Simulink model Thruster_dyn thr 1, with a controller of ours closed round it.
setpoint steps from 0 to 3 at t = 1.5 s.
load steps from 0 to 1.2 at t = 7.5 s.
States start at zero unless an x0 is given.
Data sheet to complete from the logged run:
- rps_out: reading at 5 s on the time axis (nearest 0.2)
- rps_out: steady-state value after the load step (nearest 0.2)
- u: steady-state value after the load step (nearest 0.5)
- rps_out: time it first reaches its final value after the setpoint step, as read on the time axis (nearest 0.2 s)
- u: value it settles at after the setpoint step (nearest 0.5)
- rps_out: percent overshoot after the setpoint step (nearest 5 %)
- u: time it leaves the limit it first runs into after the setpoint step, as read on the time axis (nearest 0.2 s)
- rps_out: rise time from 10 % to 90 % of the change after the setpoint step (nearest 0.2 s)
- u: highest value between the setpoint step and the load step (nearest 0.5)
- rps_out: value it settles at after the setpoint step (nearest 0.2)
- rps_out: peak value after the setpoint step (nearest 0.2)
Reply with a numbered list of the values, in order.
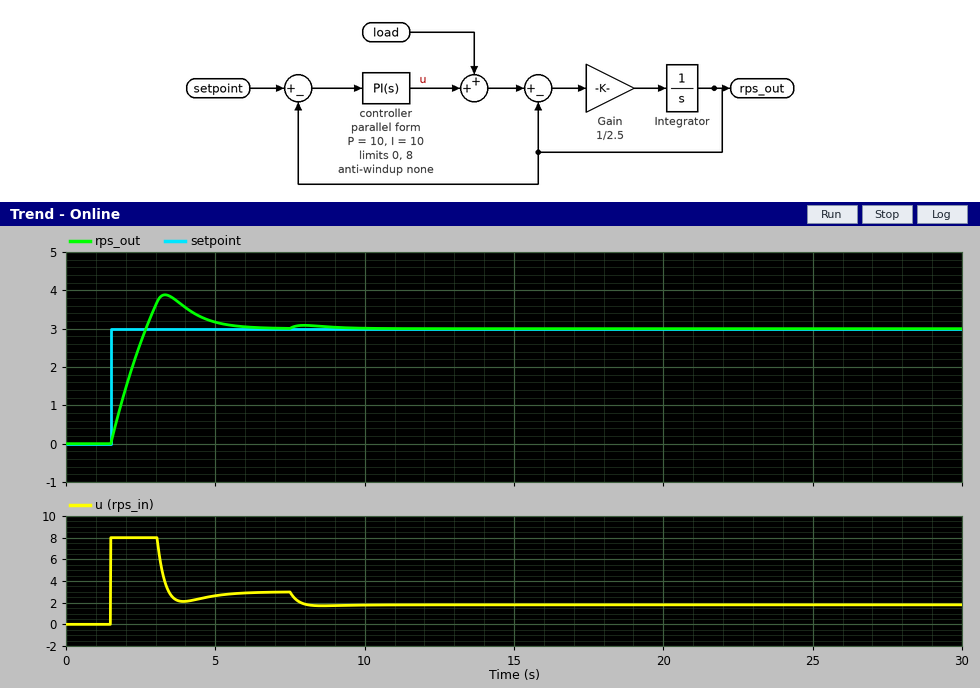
1. 3.2
2. 3.0
3. 2.0
4. 2.6 s
5. 3.0
6. 30 %
7. 3.0 s
8. 1.0 s
9. 8.0
10. 3.0
11. 3.8
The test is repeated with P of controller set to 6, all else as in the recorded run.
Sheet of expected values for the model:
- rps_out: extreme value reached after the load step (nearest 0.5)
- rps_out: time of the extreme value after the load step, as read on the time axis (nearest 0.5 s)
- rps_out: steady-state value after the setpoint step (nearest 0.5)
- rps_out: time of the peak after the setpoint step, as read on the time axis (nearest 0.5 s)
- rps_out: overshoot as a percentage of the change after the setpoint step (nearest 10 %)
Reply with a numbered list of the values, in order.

1. 3.0
2. 8.0 s
3. 3.0
4. 3.5 s
5. 40 %
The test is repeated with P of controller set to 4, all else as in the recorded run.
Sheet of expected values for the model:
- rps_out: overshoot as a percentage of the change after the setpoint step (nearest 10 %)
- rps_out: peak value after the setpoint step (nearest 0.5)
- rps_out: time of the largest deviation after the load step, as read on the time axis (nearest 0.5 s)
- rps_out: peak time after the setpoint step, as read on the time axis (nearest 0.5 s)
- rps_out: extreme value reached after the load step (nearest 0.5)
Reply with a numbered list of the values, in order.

1. 40 %
2. 4.5
3. 10.0 s
4. 3.5 s
5. 3.0
